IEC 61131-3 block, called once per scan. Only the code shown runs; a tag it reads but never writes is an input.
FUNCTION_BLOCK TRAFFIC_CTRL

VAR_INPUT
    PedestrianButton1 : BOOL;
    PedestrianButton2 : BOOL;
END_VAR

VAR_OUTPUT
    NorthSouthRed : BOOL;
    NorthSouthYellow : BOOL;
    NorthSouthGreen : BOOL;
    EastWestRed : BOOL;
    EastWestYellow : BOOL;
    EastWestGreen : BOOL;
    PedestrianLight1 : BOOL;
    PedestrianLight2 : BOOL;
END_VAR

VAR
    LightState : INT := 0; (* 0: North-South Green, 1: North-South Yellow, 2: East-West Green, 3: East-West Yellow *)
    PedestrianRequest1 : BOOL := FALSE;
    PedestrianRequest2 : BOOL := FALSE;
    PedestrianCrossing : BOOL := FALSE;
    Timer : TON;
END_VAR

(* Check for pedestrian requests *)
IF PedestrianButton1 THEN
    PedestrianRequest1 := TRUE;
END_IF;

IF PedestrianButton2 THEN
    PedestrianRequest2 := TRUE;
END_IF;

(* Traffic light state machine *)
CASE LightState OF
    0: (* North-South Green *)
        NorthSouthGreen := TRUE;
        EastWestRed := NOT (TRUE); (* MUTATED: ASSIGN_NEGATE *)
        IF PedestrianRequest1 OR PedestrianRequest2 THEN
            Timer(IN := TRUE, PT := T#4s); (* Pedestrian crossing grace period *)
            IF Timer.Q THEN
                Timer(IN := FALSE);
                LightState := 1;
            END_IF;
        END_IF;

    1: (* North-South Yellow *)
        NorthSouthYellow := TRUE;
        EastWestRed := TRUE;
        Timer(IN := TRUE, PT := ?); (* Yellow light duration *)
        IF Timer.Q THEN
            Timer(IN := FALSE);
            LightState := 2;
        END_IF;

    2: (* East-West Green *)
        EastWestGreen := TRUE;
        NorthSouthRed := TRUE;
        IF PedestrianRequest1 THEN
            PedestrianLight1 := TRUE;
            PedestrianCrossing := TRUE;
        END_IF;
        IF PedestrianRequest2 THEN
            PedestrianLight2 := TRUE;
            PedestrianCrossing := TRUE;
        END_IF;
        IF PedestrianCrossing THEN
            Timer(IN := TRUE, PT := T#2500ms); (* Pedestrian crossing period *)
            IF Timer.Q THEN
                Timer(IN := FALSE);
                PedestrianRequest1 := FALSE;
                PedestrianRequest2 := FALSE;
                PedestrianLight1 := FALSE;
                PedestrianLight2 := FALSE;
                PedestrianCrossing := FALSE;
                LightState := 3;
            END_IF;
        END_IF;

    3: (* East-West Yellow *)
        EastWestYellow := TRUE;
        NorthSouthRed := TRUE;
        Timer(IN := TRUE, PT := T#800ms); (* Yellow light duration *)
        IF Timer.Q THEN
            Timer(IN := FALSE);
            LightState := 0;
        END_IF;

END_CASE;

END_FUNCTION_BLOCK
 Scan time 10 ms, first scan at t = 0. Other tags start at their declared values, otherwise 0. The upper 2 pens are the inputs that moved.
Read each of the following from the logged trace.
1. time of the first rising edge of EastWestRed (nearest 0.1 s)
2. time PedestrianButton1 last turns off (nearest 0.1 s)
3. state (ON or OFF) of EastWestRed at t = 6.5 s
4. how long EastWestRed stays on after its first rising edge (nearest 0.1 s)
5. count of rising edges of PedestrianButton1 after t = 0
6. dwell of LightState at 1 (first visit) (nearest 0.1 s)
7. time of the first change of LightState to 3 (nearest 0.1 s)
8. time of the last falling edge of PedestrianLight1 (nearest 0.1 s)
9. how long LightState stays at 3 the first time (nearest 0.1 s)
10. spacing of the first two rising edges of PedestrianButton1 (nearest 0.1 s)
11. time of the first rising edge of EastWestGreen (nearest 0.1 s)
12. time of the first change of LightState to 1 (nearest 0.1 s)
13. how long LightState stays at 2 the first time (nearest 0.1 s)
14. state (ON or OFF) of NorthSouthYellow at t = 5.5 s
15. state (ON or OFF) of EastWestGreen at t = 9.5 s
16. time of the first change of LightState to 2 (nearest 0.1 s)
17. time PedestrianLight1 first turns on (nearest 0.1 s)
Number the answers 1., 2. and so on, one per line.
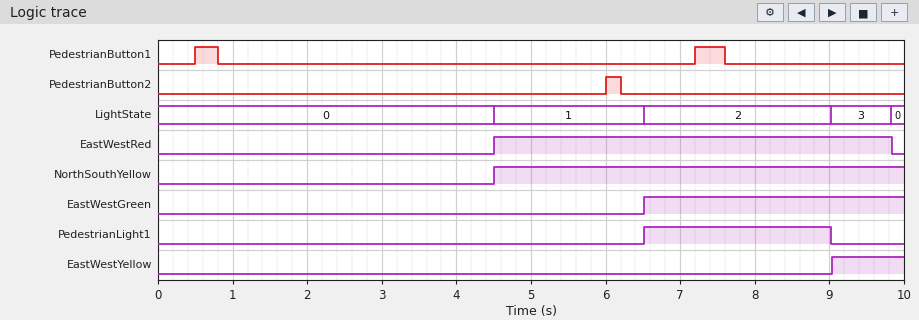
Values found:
1. 4.5 s
2. 7.6 s
3. ON
4. 5.3 s
5. 2
6. 2.0 s
7. 9.0 s
8. 9.0 s
9. 0.8 s
10. 6.7 s
11. 6.5 s
12. 4.5 s
13. 2.5 s
14. ON
15. ON
16. 6.5 s
17. 6.5 s
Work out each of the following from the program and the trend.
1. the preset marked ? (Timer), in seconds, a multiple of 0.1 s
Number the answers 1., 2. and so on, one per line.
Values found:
1. 2.0 s
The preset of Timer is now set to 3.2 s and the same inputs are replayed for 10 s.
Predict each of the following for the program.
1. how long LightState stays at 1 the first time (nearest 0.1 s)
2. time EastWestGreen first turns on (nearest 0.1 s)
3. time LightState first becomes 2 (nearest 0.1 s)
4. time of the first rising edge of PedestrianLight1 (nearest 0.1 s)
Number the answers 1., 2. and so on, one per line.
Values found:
1. 3.2 s
2. 7.7 s
3. 7.7 s
4. 7.7 s
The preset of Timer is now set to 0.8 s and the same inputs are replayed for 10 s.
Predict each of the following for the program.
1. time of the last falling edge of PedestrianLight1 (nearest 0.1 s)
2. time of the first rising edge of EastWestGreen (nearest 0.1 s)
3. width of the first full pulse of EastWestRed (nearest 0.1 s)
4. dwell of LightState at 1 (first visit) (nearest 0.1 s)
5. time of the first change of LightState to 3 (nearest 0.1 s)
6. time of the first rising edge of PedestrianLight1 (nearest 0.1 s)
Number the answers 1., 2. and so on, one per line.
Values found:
1. 7.8 s
2. 5.3 s
3. 4.1 s
4. 0.8 s
5. 7.8 s
6. 5.3 s
